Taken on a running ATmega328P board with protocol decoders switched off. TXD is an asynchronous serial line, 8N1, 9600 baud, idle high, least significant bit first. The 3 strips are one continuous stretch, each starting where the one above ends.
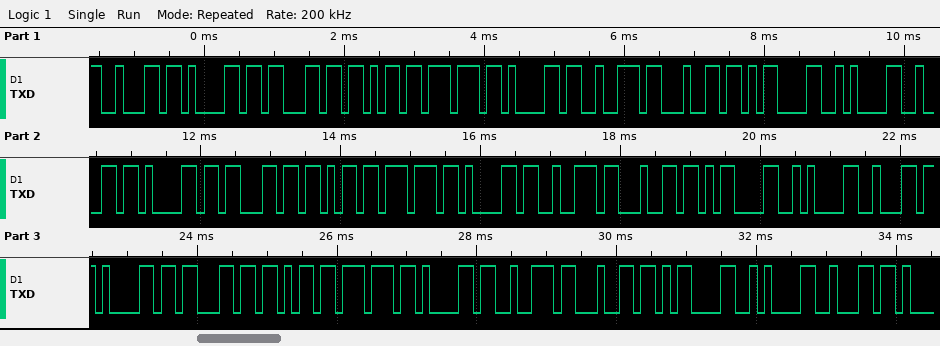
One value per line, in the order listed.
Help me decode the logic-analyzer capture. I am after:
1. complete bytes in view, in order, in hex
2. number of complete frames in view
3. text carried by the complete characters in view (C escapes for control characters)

62 61 63 6B 77 61 72 64 0D 0A 62 61 63 6B 77 61 72 64 0D 0A 62 61 63 6B 77 61 72 64 0D 0A 62
31
"backward\r\nbackward\r\nbackward\r\nb"
